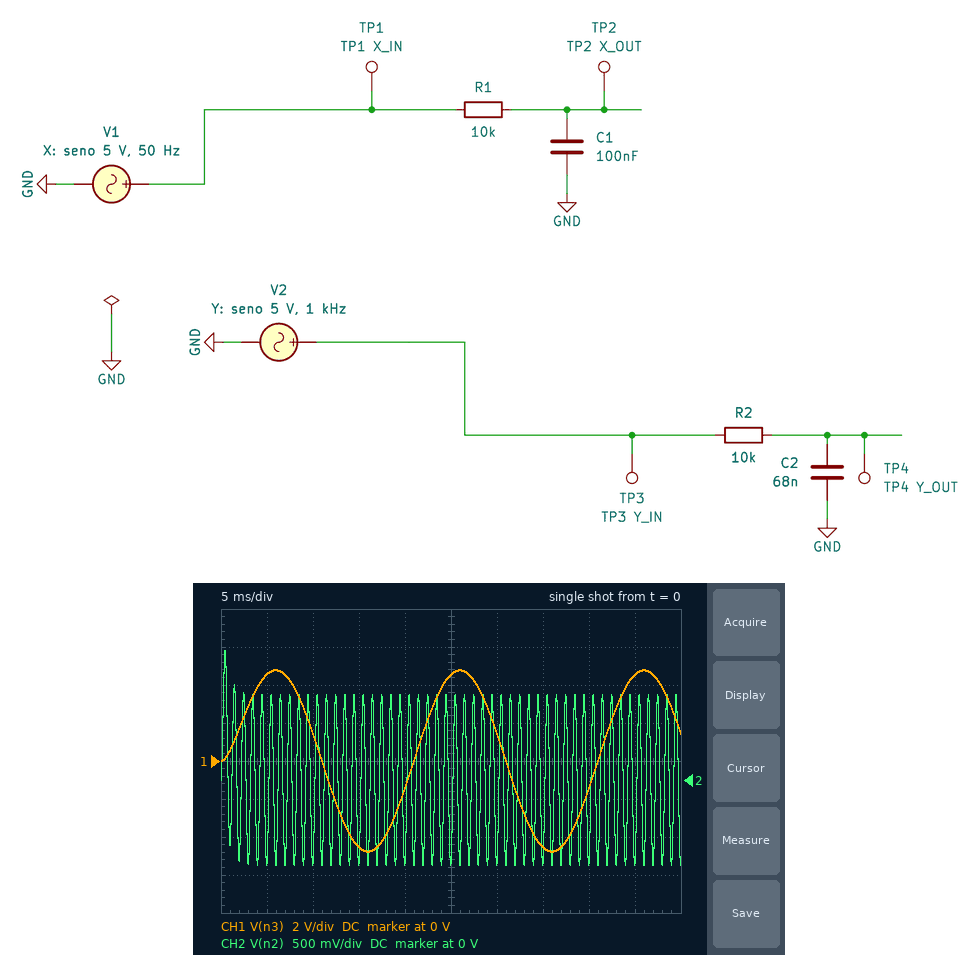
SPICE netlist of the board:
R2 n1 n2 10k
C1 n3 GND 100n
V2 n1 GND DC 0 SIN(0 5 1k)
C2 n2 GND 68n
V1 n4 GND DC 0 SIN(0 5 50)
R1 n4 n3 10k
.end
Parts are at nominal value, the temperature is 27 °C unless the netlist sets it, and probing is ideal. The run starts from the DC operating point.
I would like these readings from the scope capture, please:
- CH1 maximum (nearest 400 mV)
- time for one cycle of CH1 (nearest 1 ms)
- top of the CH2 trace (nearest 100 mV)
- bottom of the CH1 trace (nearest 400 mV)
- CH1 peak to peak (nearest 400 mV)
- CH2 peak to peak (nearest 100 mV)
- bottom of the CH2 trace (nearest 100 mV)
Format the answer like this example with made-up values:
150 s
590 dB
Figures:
4.8 V
20 ms
1.7 V
-4.8 V
9.6 V
2.8 V
-1.1 V
